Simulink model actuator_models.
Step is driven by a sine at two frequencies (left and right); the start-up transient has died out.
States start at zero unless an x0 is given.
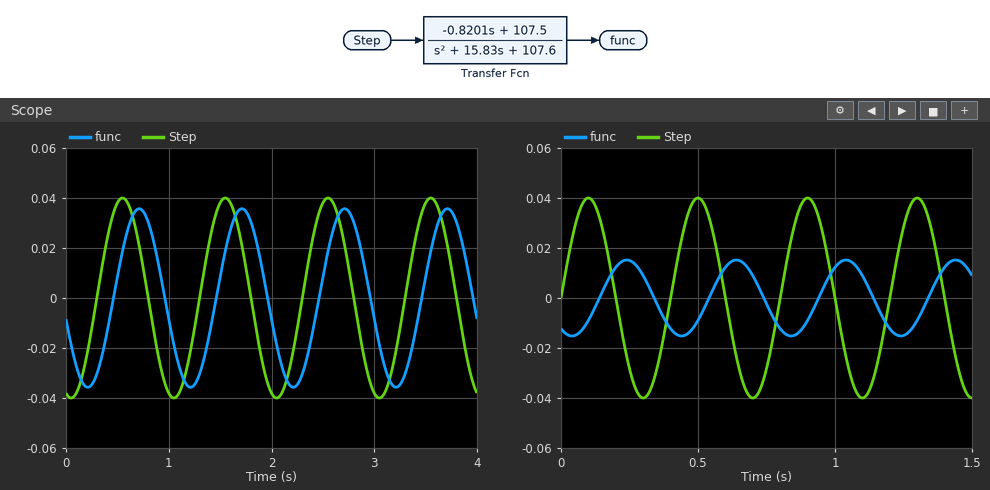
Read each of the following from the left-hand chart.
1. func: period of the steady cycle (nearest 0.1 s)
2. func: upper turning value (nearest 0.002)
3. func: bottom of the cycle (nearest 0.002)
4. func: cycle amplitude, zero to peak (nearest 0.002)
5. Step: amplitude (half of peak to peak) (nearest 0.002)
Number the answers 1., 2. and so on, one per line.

1. 1.0 s
2. 0.036
3. -0.036
4. 0.036
5. 0.040
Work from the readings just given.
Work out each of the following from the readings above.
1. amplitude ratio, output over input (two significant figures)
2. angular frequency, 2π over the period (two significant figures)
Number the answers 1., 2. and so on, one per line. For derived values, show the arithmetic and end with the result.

1. 0.036 / 0.04 = 0.90
2. 2π / 1 = 6.3 rad/s
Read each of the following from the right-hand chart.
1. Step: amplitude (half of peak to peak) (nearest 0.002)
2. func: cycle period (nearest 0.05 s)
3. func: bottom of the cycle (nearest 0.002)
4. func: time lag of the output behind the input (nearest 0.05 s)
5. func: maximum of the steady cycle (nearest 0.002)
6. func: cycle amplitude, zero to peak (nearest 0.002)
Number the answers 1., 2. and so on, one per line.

1. 0.040
2. 0.40 s
3. -0.016
4. 0.15 s
5. 0.016
6. 0.016
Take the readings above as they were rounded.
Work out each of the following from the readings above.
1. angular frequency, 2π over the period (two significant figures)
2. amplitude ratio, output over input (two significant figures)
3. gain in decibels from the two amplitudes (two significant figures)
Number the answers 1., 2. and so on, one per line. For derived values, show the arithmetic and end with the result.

1. 2π / 0.4 = 16 rad/s
2. 0.016 / 0.04 = 0.40
3. 20 log10(0.016 / 0.04) = -8.0 dB
